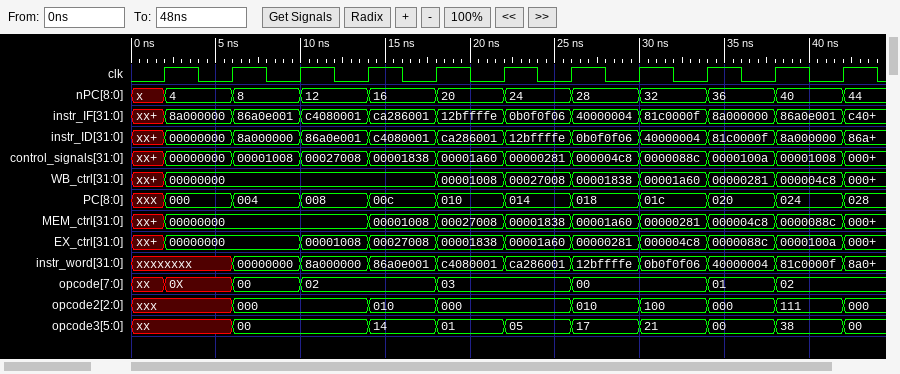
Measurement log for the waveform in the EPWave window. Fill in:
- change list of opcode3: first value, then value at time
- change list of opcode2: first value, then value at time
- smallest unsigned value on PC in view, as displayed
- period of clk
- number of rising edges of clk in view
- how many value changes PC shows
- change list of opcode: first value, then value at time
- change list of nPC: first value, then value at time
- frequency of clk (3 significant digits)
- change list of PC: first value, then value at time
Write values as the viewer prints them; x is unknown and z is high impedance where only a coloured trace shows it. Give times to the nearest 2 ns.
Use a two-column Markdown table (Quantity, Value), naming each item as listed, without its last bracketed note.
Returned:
| Quantity | Value |
|---|---|
| change list of opcode3: first value, then value at time | xx, 00 at 6 ns, 14 at 14 ns, 01 at 18 ns, 05 at 22 ns, 17 at 26 ns, 21 at 30 ns, 00 at 34 ns, 38 at 38 ns, 00 at 42 ns |
| change list of opcode2: first value, then value at time | xxx, 000 at 6 ns, 010 at 14 ns, 000 at 18 ns, 010 at 26 ns, 100 at 30 ns, 000 at 34 ns, 111 at 38 ns, 000 at 42 ns |
| smallest unsigned value on PC in view, as displayed | 000 |
| period of clk | 4 ns |
| number of rising edges of clk in view | 11 |
| how many value changes PC shows | 11 |
| change list of opcode: first value, then value at time | xx, 0X at 2 ns, 00 at 6 ns, 02 at 10 ns, 03 at 18 ns, 00 at 26 ns, 01 at 34 ns, 02 at 38 ns |
| change list of nPC: first value, then value at time | x, 4 at 2 ns, 8 at 6 ns, 12 at 10 ns, 16 at 14 ns, 20 at 18 ns, 24 at 22 ns, 28 at 26 ns, 32 at 30 ns, 36 at 34 ns, 40 at 38 ns, 44 at 42 ns |
| frequency of clk | 250 MHz |
| change list of PC: first value, then value at time | xxx, 000 at 2 ns, 004 at 6 ns, 008 at 10 ns, 00c at 14 ns, 010 at 18 ns, 014 at 22 ns, 018 at 26 ns, 01c at 30 ns, 020 at 34 ns, 024 at 38 ns, 028 at 42 ns |
